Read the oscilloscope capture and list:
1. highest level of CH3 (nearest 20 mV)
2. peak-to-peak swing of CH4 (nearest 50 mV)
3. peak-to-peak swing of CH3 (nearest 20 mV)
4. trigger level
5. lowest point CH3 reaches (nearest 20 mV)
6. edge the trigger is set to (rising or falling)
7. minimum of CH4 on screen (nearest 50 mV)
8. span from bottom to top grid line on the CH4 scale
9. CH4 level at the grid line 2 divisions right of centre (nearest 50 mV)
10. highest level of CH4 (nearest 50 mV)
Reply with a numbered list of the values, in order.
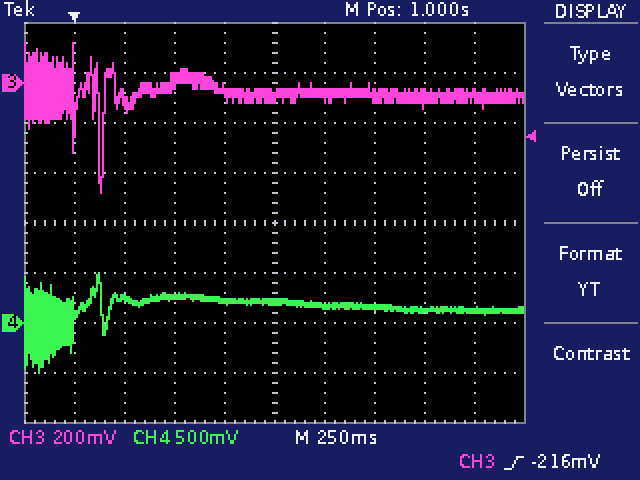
1. 160 mV
2. 1.00 V
3. 600 mV
4. -216 mV
5. -440 mV
6. rising
7. -500 mV
8. 4 V
9. 150 mV
10. 500 mV
